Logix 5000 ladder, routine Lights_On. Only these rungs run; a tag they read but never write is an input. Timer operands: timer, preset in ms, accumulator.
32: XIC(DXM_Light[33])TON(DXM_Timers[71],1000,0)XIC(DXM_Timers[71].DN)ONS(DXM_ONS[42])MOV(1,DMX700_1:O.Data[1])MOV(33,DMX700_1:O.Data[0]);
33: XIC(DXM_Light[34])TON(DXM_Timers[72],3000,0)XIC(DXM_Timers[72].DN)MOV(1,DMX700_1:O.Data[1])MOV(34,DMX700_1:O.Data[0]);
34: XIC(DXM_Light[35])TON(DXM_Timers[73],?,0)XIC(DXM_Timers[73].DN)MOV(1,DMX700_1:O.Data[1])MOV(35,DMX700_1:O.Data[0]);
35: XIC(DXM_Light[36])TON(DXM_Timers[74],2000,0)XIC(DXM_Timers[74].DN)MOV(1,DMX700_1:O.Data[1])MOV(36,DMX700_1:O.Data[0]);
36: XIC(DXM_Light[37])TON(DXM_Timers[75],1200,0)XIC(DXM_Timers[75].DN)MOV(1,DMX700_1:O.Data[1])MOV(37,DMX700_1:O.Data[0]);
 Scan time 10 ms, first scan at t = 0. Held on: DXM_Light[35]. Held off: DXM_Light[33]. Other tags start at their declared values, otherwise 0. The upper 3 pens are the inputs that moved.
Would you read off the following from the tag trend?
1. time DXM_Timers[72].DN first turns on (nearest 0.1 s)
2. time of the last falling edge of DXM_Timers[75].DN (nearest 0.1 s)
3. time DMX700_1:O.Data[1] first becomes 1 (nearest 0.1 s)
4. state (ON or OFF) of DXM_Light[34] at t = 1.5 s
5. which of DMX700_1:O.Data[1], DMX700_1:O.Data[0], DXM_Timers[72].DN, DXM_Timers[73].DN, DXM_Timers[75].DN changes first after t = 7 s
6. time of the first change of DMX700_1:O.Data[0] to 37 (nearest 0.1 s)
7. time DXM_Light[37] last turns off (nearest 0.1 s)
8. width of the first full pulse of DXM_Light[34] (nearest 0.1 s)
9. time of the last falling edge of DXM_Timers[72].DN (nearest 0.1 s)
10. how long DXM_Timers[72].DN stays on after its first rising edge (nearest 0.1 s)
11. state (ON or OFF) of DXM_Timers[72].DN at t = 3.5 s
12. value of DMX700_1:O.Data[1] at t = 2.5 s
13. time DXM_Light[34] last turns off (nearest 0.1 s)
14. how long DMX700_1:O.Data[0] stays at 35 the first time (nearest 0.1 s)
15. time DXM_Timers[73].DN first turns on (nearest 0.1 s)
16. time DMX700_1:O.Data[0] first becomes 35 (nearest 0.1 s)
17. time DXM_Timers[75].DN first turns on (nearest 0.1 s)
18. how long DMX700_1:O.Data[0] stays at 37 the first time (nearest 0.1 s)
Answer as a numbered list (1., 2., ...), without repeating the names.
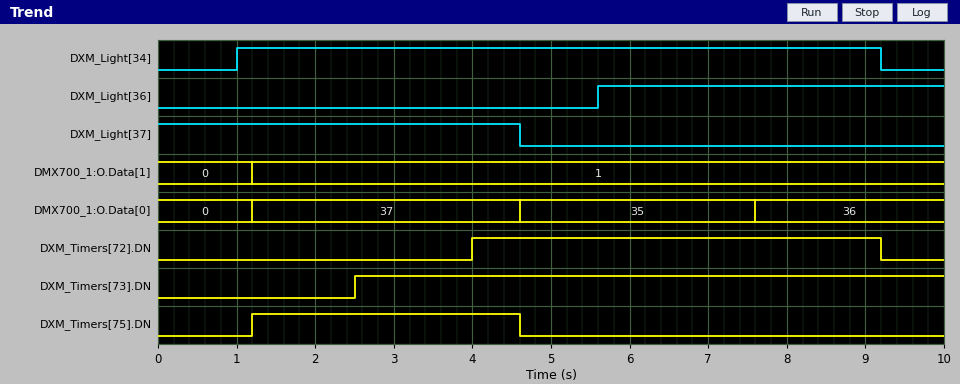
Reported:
1. 4.0 s
2. 4.6 s
3. 1.2 s
4. ON
5. DMX700_1:O.Data[0]
6. 1.2 s
7. 4.6 s
8. 8.2 s
9. 9.2 s
10. 5.2 s
11. OFF
12. 1
13. 9.2 s
14. 3.0 s
15. 2.5 s
16. 4.6 s
17. 1.2 s
18. 3.4 s
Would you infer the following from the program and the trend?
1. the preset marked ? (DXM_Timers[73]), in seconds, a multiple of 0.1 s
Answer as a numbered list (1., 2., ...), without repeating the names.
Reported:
1. 2.5 s
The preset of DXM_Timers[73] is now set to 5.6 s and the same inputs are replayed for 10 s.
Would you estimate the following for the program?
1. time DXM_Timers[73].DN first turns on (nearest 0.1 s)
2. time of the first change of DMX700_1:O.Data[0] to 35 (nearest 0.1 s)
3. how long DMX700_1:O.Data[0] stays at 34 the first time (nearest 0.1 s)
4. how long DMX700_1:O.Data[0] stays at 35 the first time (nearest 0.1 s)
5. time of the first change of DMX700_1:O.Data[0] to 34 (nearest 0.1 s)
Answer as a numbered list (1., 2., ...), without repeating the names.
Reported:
1. 5.6 s
2. 5.6 s
3. 1.0 s
4. 2.0 s
5. 4.6 s
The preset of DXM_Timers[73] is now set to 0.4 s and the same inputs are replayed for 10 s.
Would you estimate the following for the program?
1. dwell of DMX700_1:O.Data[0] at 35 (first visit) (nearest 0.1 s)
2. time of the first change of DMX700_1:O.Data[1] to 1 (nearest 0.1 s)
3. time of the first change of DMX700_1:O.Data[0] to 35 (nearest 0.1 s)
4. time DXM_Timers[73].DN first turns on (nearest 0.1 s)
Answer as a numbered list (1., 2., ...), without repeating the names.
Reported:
1. 0.8 s
2. 0.4 s
3. 0.4 s
4. 0.4 s
